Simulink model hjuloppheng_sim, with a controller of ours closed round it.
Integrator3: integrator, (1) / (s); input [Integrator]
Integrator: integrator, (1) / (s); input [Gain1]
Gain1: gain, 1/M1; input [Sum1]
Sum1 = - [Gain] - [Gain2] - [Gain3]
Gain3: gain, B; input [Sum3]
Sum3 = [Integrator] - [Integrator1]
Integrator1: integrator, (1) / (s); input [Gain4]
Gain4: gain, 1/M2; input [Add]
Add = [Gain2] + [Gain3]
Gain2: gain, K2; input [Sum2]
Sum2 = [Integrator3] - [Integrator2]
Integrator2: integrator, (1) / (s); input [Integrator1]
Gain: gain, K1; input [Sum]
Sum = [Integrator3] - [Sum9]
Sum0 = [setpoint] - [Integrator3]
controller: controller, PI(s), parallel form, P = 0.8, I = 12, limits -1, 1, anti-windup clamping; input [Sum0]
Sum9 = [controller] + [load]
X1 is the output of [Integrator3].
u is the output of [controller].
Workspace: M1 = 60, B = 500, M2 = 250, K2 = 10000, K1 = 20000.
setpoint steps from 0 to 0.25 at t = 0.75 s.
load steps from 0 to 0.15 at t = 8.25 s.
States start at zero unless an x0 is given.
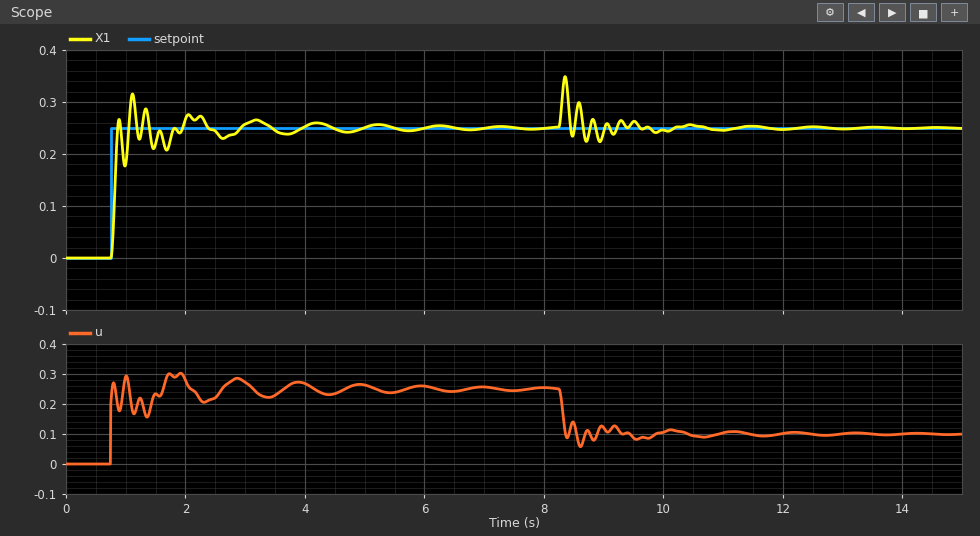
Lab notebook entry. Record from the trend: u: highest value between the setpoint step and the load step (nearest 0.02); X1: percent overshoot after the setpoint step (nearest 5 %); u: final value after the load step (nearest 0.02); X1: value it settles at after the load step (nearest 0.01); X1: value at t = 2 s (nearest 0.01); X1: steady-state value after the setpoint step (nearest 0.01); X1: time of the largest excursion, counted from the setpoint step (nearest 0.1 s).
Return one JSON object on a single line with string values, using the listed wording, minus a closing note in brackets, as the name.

{"u: highest value between the setpoint step and the load step": "0.30", "X1: percent overshoot after the setpoint step": "25 %", "u: final value after the load step": "0.10", "X1: value it settles at after the load step": "0.25", "X1: value at t = 2 s": "0.27", "X1: steady-state value after the setpoint step": "0.25", "X1: time of the largest excursion, counted from the setpoint step": "0.4 s"}
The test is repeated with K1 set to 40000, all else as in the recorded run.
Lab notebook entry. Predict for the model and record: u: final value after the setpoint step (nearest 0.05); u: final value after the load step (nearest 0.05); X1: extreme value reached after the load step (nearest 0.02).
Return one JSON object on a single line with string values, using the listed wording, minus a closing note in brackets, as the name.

{"u: final value after the setpoint step": "0.25", "u: final value after the load step": "0.10", "X1: extreme value reached after the load step": "0.36"}
